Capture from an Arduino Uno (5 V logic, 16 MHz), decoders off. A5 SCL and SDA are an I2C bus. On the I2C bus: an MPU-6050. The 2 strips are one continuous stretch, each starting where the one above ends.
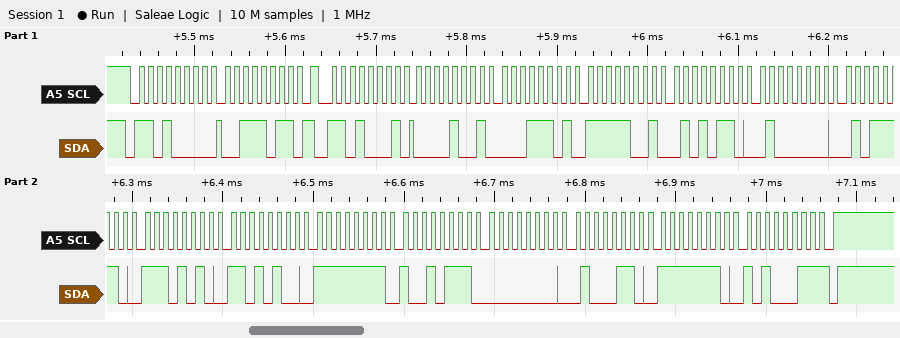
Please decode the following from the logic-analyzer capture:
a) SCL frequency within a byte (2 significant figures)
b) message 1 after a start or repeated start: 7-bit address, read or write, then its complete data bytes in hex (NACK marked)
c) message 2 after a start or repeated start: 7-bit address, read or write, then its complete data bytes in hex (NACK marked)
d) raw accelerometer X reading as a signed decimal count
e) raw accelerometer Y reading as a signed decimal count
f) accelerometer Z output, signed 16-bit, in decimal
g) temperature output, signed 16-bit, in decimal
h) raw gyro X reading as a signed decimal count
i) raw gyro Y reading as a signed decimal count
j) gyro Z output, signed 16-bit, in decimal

100 kHz
0x68 write: 3B
0x68 read: 09 1D F9 56 40 5E EA D4 FF 97 00 46 FE A3 NACK
2333
-1706
16478
-5420
-105
70
-349
